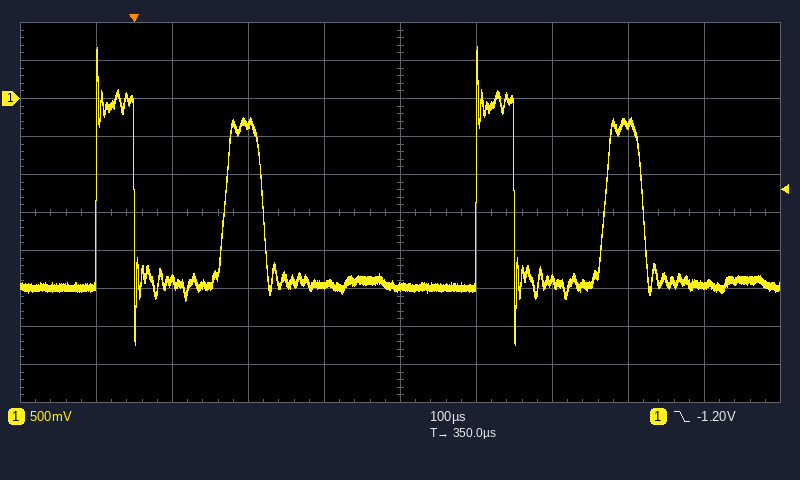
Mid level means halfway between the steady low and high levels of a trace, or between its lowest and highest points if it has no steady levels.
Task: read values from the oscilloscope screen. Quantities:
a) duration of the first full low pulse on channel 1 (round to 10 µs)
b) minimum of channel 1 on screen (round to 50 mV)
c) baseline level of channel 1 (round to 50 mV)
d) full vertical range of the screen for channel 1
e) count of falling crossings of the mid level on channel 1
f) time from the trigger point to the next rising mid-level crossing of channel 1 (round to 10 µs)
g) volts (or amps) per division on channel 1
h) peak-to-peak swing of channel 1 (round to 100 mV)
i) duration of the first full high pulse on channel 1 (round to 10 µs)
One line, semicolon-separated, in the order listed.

120 µs; -3.25 V; -2.45 V; 5 V; 4; 120 µs; 500 mV; 3.90 V; 50 µs
